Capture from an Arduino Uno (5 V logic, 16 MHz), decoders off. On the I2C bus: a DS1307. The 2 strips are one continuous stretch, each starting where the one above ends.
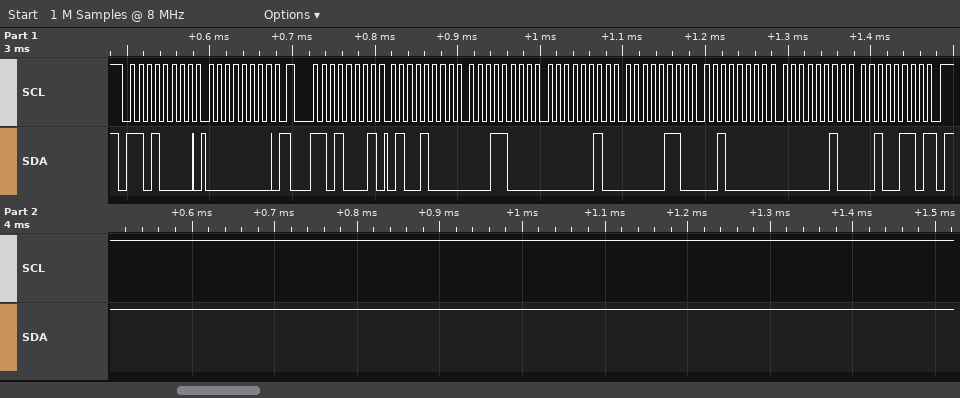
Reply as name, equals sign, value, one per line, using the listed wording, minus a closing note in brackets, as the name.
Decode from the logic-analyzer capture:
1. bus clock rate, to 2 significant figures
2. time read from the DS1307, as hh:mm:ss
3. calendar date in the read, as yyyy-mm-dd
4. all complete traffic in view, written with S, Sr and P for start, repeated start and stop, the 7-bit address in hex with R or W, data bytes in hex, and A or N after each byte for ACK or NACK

bus clock rate, to 2 significant figures = 100 kHz
time read from the DS1307, as hh:mm:ss = 02:18:48
calendar date in the read, as yyyy-mm-dd = 2026-02-20
all complete traffic in view, written with S, Sr and P for start, repeated start and stop, the 7-bit address in hex with R or W, data bytes in hex, and A or N after each byte for ACK or NACK = S 68W A 00 A Sr 68R A 48 A 18 A 02 A 06 A 20 A 02 A 26 N P
